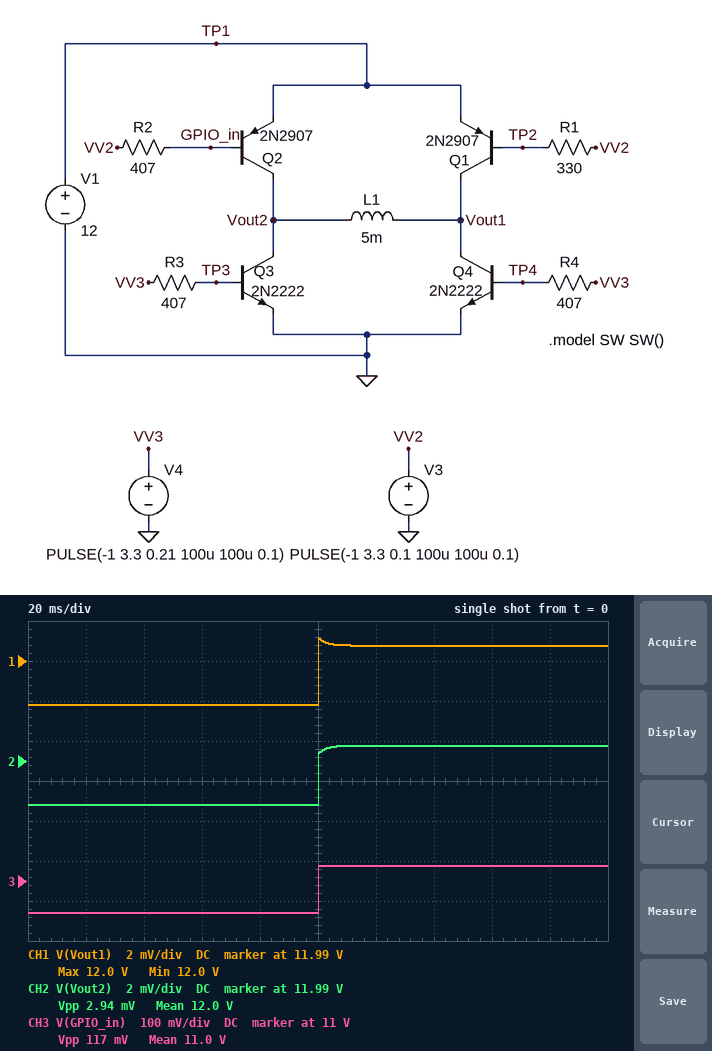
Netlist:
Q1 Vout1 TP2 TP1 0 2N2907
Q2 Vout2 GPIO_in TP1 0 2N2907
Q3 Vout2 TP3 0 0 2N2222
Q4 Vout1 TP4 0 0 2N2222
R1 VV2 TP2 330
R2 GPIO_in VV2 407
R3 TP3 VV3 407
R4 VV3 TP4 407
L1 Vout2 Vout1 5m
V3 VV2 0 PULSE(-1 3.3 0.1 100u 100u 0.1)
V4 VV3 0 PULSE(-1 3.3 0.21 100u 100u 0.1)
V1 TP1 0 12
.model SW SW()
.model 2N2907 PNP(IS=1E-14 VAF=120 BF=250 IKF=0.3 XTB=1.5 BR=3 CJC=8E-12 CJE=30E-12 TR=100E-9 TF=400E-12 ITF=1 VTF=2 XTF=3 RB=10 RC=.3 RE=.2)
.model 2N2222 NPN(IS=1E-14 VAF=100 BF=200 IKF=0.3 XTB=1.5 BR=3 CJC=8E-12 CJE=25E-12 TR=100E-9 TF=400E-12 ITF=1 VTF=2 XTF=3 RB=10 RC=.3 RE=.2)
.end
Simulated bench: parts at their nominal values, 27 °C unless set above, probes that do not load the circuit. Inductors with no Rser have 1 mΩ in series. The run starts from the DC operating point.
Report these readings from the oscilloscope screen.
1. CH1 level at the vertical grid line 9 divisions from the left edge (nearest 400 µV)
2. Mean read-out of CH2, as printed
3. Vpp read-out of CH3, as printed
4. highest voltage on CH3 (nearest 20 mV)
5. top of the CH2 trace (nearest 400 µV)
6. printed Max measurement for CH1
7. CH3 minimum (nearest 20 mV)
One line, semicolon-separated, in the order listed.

11.9868 V; 12.0 V; 117 mV; 11.04 V; 11.9868 V; 12.0 V; 10.92 V
